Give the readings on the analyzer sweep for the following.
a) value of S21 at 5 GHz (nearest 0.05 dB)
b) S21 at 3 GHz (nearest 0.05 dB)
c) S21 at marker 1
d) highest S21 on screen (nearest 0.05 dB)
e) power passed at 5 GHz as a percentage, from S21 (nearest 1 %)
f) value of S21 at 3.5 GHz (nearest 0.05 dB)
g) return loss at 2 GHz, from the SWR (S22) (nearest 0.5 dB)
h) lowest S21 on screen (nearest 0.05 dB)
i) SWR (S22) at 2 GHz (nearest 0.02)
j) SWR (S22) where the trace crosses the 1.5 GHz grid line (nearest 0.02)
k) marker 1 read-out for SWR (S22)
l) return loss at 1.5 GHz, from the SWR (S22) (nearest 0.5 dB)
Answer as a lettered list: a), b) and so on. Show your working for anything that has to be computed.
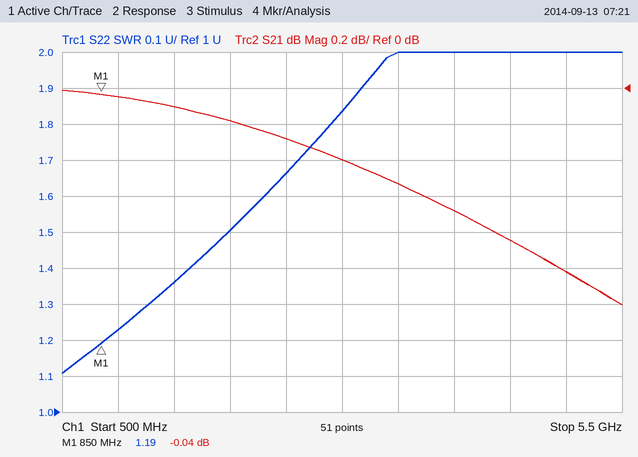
a) -1.00 dB
b) -0.40 dB
c) -0.04 dB
d) 0.00 dB
e) 10^(-1/10) ≈ 79 %
f) -0.55 dB
g) −20 log10((1.5 − 1)/(1.5 + 1)) ≈ 14.0 dB
h) -1.20 dB
i) 1.50
j) 1.36
k) 1.19
l) −20 log10((1.36 − 1)/(1.36 + 1)) ≈ 16.3 dB, so 16.5 dB to the nearest 0.5 dB
